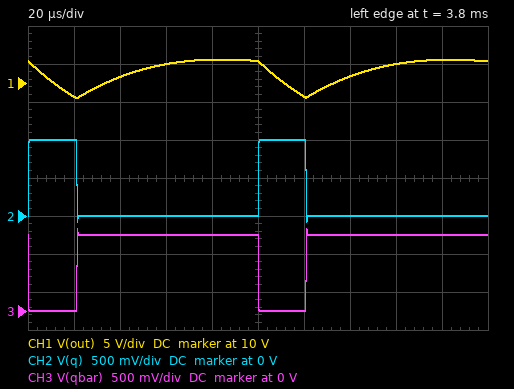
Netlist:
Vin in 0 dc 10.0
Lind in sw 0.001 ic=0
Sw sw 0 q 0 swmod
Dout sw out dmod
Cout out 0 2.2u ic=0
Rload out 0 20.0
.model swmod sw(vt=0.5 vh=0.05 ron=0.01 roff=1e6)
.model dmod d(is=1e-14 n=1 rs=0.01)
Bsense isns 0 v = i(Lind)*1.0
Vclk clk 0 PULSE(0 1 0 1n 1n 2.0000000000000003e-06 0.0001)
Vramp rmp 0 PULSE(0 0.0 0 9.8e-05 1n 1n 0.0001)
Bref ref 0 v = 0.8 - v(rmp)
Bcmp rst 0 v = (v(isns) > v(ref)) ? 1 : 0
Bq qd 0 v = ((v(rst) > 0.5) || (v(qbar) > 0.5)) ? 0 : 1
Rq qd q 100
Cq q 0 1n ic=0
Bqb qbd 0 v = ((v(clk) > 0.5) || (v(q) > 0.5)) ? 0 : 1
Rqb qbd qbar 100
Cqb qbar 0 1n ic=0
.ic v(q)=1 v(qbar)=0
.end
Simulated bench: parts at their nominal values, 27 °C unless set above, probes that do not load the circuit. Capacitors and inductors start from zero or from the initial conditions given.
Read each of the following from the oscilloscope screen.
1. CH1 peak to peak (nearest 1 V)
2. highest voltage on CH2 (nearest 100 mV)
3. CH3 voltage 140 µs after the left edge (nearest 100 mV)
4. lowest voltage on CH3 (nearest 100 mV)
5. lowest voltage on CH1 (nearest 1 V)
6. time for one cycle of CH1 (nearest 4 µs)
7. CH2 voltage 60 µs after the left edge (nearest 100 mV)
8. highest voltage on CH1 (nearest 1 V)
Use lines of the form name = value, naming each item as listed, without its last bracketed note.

CH1 peak to peak = 5 V
highest voltage on CH2 = 1.0 V
CH3 voltage 140 µs after the left edge = 1.0 V
lowest voltage on CH3 = 0 V
lowest voltage on CH1 = 8 V
time for one cycle of CH1 = 100 µs
CH2 voltage 60 µs after the left edge = 0 V
highest voltage on CH1 = 13 V
